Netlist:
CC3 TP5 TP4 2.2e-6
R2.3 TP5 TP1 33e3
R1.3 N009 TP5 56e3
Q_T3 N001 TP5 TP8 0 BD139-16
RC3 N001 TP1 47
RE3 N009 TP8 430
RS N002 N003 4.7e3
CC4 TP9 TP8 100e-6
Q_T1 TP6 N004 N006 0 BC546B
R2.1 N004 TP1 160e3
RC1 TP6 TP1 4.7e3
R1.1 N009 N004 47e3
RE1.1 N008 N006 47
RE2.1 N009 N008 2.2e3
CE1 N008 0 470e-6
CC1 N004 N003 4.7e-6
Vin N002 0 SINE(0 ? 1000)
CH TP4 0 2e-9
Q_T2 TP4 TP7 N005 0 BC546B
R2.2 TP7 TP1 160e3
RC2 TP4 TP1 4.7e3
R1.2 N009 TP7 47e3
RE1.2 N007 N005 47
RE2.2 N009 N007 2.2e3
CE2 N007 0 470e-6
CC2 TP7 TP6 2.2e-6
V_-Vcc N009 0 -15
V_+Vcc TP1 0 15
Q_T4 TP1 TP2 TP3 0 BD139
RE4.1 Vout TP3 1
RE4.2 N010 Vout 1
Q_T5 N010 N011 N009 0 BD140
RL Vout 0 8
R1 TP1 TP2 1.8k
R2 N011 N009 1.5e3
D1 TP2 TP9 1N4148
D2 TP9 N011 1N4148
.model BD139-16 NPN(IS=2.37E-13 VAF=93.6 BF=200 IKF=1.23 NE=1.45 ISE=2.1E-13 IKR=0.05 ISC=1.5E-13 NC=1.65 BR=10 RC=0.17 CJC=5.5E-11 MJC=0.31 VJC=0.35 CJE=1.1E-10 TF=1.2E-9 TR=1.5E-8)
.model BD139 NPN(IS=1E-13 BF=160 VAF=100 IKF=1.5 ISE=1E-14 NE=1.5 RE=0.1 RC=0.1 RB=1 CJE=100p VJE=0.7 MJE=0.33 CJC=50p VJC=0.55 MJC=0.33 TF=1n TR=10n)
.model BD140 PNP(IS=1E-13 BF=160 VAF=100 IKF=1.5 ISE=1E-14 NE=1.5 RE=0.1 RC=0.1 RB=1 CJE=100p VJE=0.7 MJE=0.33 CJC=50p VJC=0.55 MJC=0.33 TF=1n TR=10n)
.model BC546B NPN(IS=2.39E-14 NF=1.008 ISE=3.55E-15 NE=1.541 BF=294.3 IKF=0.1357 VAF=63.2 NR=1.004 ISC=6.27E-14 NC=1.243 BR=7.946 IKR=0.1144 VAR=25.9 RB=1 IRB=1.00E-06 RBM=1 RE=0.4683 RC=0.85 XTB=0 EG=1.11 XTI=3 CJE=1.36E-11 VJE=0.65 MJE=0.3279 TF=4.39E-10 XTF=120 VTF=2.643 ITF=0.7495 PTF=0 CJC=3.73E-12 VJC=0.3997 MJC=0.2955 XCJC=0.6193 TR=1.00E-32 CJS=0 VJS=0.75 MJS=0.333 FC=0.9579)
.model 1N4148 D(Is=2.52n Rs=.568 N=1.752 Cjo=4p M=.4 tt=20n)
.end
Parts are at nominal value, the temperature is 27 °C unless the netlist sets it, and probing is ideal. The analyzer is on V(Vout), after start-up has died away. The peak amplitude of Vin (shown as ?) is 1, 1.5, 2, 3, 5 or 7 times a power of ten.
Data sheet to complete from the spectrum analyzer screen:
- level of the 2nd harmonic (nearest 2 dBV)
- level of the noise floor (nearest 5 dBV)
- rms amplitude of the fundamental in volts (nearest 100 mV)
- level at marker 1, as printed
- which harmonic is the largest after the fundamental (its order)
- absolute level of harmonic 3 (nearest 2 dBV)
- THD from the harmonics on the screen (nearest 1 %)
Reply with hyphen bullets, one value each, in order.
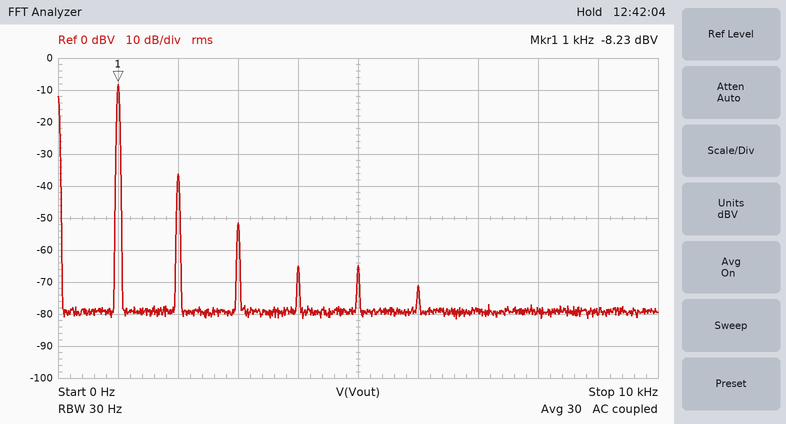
- -36 dBV
- -80 dBV
- 400 mV
- -8.23 dBV
- 2
- -52 dBV
- 4 %
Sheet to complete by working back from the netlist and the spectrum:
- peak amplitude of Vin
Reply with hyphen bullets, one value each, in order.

- 300 µV
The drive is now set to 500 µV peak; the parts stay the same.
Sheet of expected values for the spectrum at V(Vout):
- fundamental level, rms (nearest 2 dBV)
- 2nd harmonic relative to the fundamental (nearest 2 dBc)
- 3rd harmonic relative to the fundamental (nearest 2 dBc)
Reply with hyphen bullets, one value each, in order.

- -4 dBV
- -22 dBc
- -30 dBc
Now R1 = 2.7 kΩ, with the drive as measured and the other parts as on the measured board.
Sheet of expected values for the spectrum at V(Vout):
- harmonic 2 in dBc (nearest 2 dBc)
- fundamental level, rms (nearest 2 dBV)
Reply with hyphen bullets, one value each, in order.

- -14 dBc
- -10 dBV
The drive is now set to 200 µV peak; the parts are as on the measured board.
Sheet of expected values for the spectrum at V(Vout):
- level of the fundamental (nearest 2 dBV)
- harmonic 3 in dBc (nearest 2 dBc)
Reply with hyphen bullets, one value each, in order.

- -12 dBV
- -56 dBc
